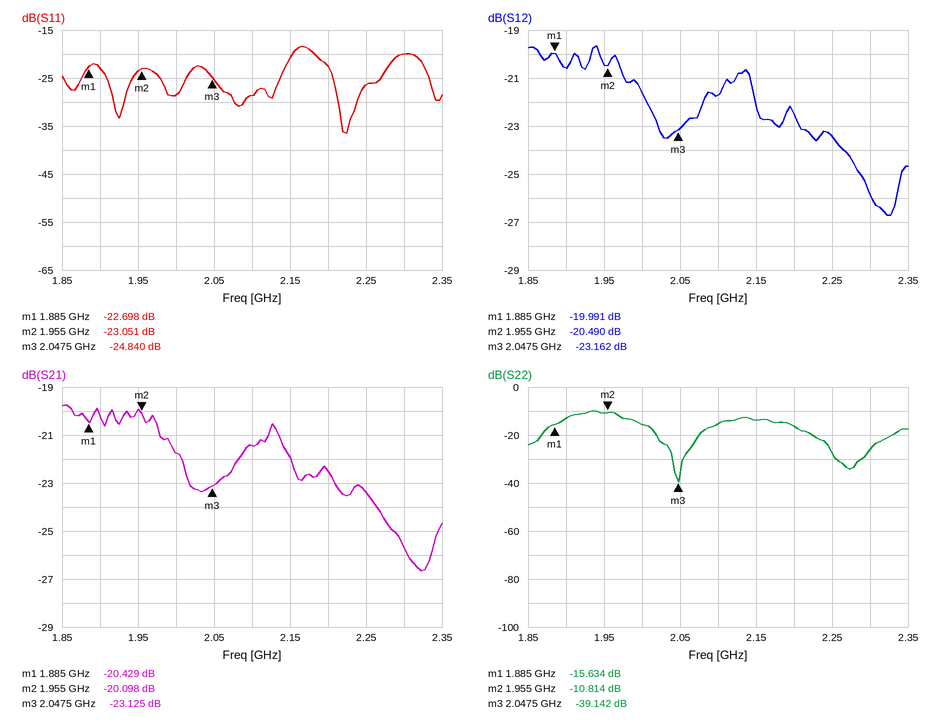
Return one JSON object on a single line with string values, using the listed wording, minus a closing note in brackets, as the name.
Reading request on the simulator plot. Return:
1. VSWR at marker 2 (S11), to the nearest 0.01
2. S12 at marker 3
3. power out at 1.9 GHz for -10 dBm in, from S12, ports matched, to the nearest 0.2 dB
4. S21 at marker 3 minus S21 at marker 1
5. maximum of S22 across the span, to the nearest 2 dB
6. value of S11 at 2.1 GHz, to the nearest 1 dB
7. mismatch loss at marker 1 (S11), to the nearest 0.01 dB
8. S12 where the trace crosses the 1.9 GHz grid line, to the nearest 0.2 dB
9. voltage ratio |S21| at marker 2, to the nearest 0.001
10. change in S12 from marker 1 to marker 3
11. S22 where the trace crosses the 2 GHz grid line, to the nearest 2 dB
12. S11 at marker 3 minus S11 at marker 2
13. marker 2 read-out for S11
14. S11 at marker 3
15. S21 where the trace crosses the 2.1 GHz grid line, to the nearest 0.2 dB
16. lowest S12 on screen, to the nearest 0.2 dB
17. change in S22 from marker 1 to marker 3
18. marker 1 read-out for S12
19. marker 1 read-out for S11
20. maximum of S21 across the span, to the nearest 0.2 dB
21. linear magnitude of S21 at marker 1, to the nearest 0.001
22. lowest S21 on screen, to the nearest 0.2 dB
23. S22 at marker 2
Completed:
{"VSWR at marker 2 (S11), to the nearest 0.01": "1.15", "S12 at marker 3": "-23.162 dB", "power out at 1.9 GHz for -10 dBm in, from S12, ports matched, to the nearest 0.2 dB": "-30.6 dBm", "S21 at marker 3 minus S21 at marker 1": "-2.696 dB", "maximum of S22 across the span, to the nearest 2 dB": "-10 dB", "value of S11 at 2.1 GHz, to the nearest 1 dB": "-29 dB", "mismatch loss at marker 1 (S11), to the nearest 0.01 dB": "0.02 dB", "S12 where the trace crosses the 1.9 GHz grid line, to the nearest 0.2 dB": "-20.6 dB", "voltage ratio |S21| at marker 2, to the nearest 0.001": "0.099", "change in S12 from marker 1 to marker 3": "-3.171 dB", "S22 where the trace crosses the 2 GHz grid line, to the nearest 2 dB": "-16 dB", "S11 at marker 3 minus S11 at marker 2": "-1.789 dB", "marker 2 read-out for S11": "-23.051 dB", "S11 at marker 3": "-24.840 dB", "S21 where the trace crosses the 2.1 GHz grid line, to the nearest 0.2 dB": "-21.4 dB", "lowest S12 on screen, to the nearest 0.2 dB": "-26.8 dB", "change in S22 from marker 1 to marker 3": "-23.508 dB", "marker 1 read-out for S12": "-19.991 dB", "marker 1 read-out for S11": "-22.698 dB", "maximum of S21 across the span, to the nearest 0.2 dB": "-19.8 dB", "linear magnitude of S21 at marker 1, to the nearest 0.001": "0.095", "lowest S21 on screen, to the nearest 0.2 dB": "-26.6 dB", "S22 at marker 2": "-10.814 dB"}
